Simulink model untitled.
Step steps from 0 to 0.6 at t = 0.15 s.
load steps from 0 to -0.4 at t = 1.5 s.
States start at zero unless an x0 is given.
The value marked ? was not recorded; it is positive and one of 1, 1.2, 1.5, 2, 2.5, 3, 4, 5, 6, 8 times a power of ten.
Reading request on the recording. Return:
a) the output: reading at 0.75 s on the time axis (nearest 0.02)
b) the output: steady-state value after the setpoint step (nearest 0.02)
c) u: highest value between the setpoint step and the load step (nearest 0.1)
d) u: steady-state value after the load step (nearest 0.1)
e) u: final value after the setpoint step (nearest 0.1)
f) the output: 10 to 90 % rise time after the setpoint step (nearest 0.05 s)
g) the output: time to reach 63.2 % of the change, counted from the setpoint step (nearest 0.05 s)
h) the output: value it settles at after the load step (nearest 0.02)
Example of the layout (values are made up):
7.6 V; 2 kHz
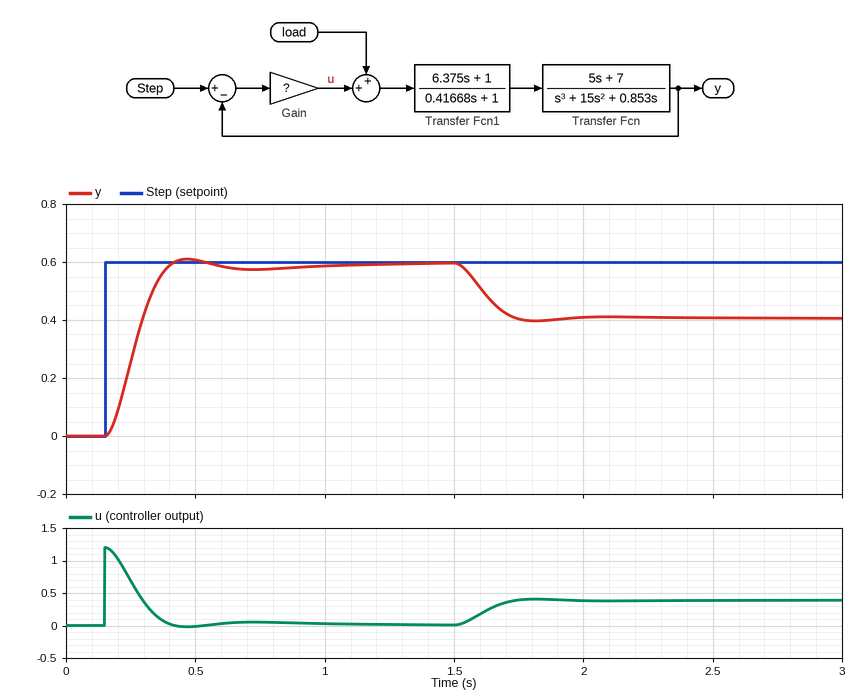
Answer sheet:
0.58; 0.60; 1.2; 0.4; 0.0; 0.15 s; 0.15 s; 0.40
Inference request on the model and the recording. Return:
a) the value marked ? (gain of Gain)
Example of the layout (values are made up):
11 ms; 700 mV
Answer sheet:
2
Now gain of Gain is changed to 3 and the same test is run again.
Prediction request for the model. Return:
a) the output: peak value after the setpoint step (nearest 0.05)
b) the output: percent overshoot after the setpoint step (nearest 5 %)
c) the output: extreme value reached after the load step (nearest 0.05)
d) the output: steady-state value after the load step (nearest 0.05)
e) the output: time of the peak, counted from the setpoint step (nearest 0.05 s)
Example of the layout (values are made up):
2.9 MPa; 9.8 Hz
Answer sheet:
0.65; 10 %; 0.45; 0.45; 0.25 s
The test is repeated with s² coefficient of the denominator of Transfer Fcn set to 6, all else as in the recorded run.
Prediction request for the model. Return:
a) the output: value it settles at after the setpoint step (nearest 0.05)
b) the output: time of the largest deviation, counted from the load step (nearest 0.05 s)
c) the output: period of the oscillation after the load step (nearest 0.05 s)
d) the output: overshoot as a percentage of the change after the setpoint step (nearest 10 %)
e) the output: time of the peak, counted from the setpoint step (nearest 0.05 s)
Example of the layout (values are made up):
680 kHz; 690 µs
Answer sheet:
0.60; 0.25 s; 0.50 s; 40 %; 0.25 s
